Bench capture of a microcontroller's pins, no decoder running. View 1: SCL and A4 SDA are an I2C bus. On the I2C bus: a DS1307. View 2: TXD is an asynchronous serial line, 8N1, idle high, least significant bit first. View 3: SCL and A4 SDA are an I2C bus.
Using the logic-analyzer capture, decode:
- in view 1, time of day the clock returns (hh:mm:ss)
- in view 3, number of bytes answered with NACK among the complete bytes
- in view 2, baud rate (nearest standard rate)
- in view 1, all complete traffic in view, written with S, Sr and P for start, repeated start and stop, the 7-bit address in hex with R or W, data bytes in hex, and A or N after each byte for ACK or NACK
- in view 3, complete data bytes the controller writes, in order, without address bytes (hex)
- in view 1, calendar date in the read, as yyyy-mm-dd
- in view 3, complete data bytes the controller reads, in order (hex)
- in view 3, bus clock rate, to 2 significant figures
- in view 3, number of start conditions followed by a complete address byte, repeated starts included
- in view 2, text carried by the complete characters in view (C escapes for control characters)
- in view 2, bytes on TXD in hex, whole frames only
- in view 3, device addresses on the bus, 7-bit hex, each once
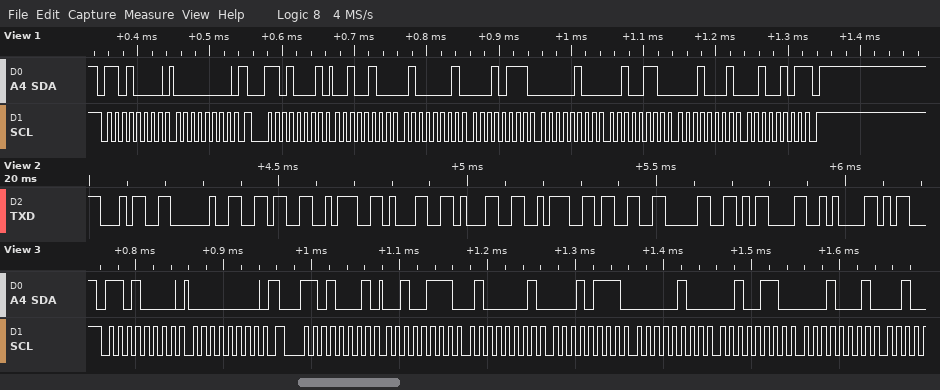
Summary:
17:41:24
0
57600 baud
S 68W A 00 A Sr 68R A 24 A 41 A 17 A 04 A 26 A 11 A 25 N P
00
2025-11-26
27 41 17 04 26 11
100 kHz
2
"4 6:11:30\r\n"
34 20 36 3A 31 31 3A 33 30 0D 0A
0x68
